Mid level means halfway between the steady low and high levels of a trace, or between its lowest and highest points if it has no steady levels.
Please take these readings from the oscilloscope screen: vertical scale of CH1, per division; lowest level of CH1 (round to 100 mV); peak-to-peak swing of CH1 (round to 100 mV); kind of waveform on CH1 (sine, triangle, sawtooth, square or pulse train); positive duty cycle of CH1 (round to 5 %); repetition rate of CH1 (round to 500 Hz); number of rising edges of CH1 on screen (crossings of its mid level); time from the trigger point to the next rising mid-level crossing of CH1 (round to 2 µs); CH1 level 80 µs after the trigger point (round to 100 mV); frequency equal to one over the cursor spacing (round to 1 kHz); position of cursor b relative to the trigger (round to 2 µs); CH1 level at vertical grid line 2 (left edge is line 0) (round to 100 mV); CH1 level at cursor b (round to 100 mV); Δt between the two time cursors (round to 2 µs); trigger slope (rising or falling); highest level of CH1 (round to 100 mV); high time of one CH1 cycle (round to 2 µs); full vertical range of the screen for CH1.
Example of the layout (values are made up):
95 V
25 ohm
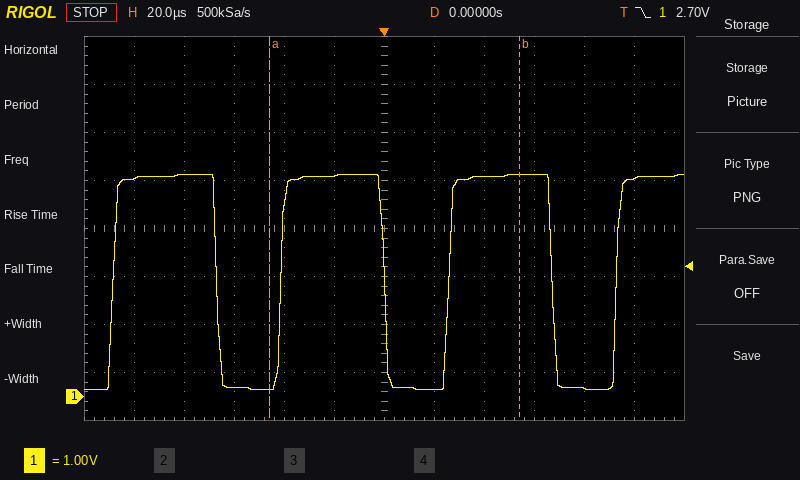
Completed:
1 V
100 mV
4.5 V
pulse train
60 %
15.0 kHz
4
26 µs
200 mV
10 kHz
+54 µs
4.6 V
4.6 V
100 µs
falling
4.6 V
42 µs
8 V
